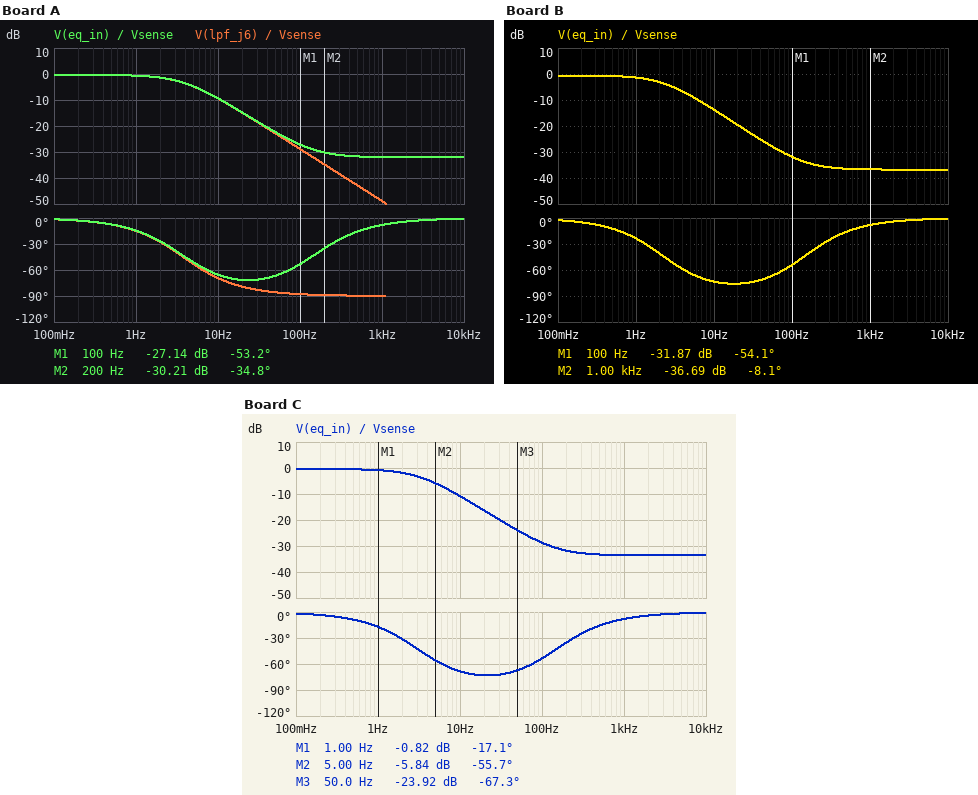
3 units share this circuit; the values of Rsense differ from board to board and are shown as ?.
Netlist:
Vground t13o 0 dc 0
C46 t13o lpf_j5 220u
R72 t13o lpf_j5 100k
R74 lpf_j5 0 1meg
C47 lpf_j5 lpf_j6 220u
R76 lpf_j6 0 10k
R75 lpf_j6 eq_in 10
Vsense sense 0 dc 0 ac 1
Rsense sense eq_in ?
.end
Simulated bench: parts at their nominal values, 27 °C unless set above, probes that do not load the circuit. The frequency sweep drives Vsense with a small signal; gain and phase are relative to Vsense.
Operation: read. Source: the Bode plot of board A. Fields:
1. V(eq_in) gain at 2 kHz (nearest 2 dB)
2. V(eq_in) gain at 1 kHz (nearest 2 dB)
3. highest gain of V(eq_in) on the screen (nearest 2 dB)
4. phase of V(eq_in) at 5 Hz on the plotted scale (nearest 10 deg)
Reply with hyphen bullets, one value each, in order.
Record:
- -32 dB
- -32 dB
- 0 dB
- -50 deg
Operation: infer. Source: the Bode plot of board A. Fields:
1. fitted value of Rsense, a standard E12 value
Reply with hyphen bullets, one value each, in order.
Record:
- 390 Ω
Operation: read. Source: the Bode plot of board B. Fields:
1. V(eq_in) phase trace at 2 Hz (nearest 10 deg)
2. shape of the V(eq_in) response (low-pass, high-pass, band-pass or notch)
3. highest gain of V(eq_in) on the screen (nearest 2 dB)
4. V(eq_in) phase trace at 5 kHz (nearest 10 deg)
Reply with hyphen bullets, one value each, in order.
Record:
- -40 deg
- low-pass
- 0 dB
- 0 deg
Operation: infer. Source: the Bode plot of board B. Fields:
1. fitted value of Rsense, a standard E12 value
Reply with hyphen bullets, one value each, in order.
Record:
- 680 Ω
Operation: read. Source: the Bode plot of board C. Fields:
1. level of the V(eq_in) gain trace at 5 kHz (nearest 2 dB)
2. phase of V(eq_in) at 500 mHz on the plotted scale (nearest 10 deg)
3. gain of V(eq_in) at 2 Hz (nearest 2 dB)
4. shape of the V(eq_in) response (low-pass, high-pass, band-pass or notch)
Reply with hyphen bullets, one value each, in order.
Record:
- -34 dB
- -10 deg
- -2 dB
- low-pass
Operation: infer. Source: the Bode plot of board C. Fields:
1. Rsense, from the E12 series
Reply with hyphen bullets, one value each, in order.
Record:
- 470 Ω
